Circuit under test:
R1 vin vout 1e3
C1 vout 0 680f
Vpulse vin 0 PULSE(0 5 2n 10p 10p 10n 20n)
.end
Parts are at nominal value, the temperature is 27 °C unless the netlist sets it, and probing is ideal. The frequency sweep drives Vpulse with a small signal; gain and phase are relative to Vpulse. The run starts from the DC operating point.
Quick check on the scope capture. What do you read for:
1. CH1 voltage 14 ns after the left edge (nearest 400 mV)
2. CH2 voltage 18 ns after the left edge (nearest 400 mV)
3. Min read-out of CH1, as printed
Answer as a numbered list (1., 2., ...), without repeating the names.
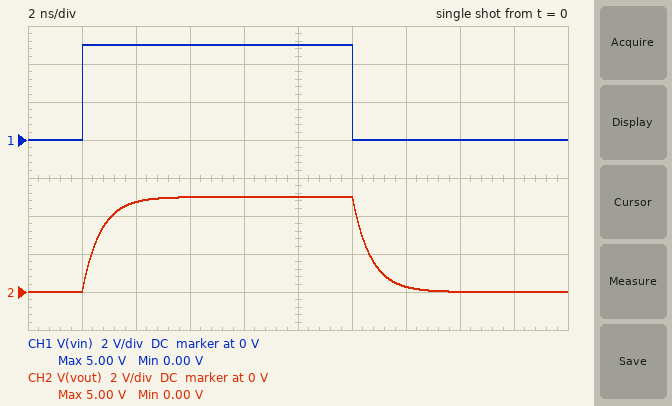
1. 0 V
2. 0 V
3. 0.00 V
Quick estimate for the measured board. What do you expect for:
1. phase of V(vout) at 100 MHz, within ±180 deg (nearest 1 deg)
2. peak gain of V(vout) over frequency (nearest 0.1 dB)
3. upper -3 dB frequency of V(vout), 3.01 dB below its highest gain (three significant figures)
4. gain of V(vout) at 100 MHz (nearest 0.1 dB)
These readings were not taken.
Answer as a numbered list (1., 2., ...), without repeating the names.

1. -23 deg
2. 0 dB
3. 234 MHz
4. -0.7 dB
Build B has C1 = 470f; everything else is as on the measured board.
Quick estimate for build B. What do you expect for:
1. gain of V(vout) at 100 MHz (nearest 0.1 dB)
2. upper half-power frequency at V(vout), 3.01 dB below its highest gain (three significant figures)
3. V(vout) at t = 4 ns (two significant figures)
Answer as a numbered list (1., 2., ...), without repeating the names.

1. -0.4 dB
2. 339 MHz
3. 4.9 V
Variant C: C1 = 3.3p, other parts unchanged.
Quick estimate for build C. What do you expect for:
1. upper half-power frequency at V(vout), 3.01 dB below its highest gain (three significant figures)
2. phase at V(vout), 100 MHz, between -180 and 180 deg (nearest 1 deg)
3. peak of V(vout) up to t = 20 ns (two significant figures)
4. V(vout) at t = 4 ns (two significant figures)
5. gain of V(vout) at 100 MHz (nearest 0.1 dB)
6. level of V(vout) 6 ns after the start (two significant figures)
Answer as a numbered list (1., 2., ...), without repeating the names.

1. 48.2 MHz
2. -64 deg
3. 4.8 V
4. 2.3 V
5. -7.2 dB
6. 3.5 V
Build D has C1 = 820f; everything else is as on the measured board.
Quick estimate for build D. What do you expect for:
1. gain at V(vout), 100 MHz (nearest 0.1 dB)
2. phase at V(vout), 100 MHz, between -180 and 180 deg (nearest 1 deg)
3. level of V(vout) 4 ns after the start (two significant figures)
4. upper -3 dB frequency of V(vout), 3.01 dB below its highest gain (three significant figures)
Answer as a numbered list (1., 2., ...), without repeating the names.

1. -1.0 dB
2. -27 deg
3. 4.6 V
4. 194 MHz
